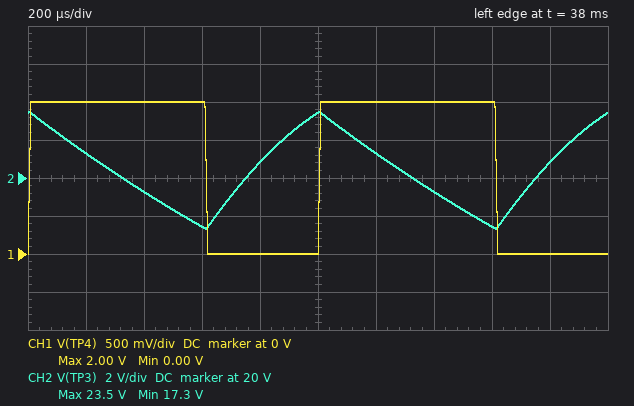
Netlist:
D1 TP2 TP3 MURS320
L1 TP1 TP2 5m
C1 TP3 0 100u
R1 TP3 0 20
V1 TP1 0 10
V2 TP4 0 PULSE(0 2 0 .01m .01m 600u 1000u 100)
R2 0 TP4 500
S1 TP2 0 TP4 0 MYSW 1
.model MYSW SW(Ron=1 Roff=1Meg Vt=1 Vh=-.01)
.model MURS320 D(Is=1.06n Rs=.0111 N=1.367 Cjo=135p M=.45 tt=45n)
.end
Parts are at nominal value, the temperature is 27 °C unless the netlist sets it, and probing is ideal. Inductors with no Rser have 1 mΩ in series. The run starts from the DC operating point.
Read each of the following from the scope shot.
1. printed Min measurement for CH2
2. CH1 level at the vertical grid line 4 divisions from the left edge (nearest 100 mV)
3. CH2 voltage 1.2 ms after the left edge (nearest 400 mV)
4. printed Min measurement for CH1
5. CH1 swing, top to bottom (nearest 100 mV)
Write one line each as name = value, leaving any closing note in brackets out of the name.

printed Min measurement for CH2 = 17.3 V
CH1 level at the vertical grid line 4 divisions from the left edge = 0 V
CH2 voltage 1.2 ms after the left edge = 21.2 V
printed Min measurement for CH1 = 0.00 V
CH1 swing, top to bottom = 2.0 V
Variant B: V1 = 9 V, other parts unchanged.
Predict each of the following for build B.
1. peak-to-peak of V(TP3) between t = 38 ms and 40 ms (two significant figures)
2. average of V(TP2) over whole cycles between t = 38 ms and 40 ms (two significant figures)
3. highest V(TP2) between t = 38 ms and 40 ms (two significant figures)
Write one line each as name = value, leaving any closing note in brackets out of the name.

peak-to-peak of V(TP3) between t = 38 ms and 40 ms = 5.5 V
average of V(TP2) over whole cycles between t = 38 ms and 40 ms = 9.0 V
highest V(TP2) between t = 38 ms and 40 ms = 22 V
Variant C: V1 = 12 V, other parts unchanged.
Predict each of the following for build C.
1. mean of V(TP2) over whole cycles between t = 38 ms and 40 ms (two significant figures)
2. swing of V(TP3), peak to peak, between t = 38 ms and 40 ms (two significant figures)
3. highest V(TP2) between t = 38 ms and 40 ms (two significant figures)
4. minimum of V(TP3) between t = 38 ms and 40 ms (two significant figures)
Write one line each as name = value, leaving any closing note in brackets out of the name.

mean of V(TP2) over whole cycles between t = 38 ms and 40 ms = 12 V
swing of V(TP3), peak to peak, between t = 38 ms and 40 ms = 7.4 V
highest V(TP2) between t = 38 ms and 40 ms = 29 V
minimum of V(TP3) between t = 38 ms and 40 ms = 21 V
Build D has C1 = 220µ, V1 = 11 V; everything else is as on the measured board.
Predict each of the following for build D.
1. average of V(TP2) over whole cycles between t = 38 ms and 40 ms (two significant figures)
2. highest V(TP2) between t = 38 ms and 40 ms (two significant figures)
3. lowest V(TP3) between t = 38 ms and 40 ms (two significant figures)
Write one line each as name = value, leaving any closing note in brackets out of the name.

average of V(TP2) over whole cycles between t = 38 ms and 40 ms = 11 V
highest V(TP2) between t = 38 ms and 40 ms = 25 V
lowest V(TP3) between t = 38 ms and 40 ms = 21 V
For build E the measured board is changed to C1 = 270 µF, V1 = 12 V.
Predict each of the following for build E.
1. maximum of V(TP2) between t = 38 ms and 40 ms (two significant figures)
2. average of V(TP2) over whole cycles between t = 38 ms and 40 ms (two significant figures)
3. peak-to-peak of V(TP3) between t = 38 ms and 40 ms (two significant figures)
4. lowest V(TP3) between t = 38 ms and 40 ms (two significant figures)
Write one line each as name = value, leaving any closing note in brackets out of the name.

maximum of V(TP2) between t = 38 ms and 40 ms = 27 V
average of V(TP2) over whole cycles between t = 38 ms and 40 ms = 12 V
peak-to-peak of V(TP3) between t = 38 ms and 40 ms = 2.8 V
lowest V(TP3) between t = 38 ms and 40 ms = 23 V
